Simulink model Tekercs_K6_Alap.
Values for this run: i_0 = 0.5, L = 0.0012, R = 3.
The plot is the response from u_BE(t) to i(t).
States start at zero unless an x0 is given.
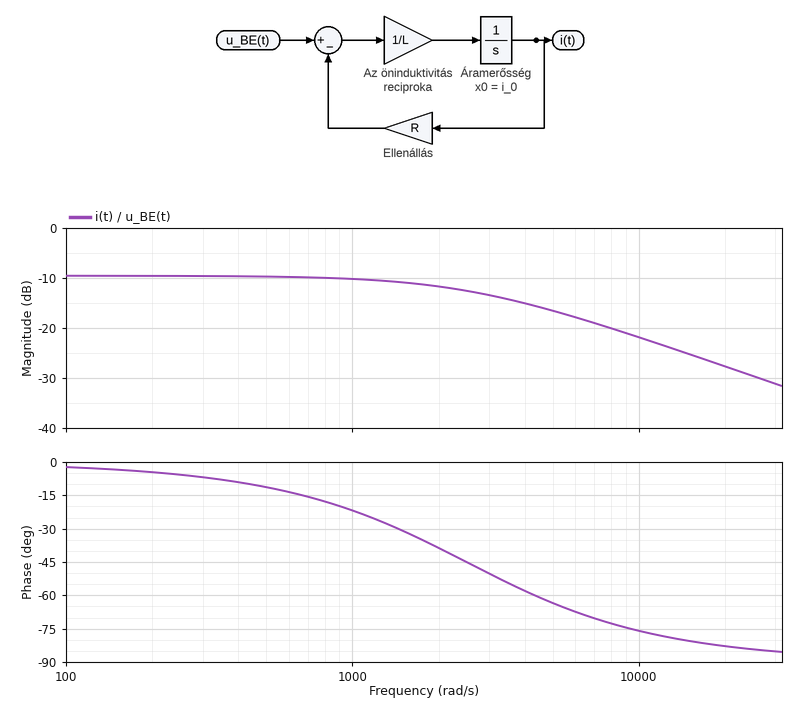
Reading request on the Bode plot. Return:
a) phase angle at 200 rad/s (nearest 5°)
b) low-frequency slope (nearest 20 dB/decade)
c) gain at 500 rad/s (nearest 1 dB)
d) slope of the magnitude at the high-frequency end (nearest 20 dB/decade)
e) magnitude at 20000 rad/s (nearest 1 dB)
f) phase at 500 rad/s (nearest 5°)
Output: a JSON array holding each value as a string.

["-5°", "0 dB/decade", "-10 dB", "-20 dB/decade", "-28 dB", "-10°"]
